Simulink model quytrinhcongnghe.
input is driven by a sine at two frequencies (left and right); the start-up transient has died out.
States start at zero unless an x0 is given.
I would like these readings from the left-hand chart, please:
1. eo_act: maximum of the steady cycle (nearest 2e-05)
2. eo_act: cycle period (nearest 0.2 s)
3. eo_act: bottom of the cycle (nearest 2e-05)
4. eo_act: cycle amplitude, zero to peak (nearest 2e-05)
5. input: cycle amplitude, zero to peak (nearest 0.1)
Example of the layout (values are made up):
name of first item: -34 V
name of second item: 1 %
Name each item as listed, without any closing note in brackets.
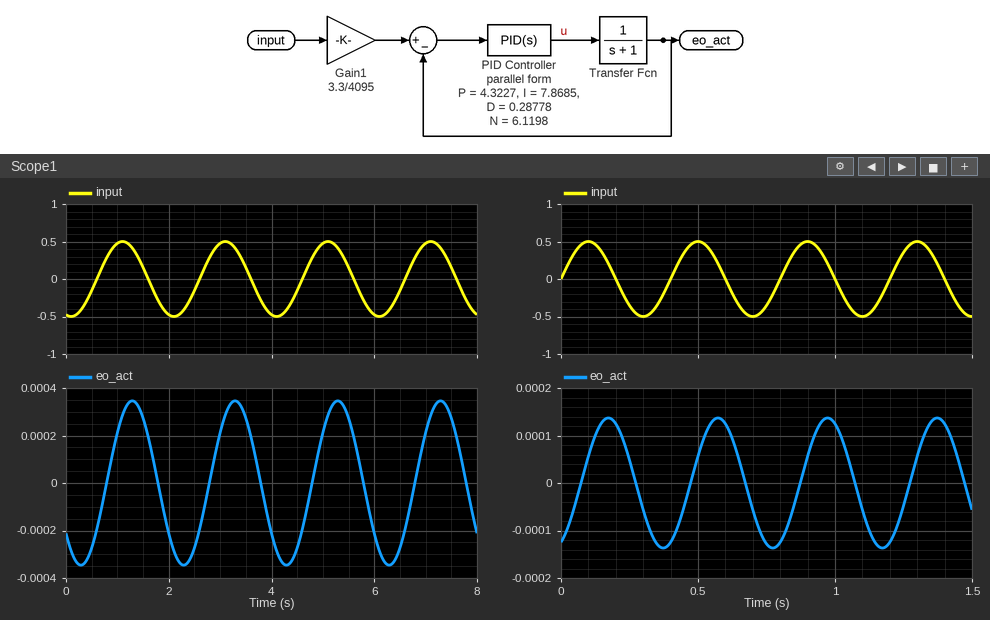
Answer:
eo_act: maximum of the steady cycle: 0.00034
eo_act: cycle period: 2.0 s
eo_act: bottom of the cycle: -0.00034
eo_act: cycle amplitude, zero to peak: 0.00034
input: cycle amplitude, zero to peak: 0.5
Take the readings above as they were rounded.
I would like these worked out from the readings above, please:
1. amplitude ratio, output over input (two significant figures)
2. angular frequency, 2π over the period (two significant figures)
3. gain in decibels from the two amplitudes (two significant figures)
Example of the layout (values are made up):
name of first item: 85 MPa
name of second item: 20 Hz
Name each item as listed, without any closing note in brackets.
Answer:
amplitude ratio, output over input: 0.00068
angular frequency, 2π over the period: 3.1 rad/s
gain in decibels from the two amplitudes: -63 dB
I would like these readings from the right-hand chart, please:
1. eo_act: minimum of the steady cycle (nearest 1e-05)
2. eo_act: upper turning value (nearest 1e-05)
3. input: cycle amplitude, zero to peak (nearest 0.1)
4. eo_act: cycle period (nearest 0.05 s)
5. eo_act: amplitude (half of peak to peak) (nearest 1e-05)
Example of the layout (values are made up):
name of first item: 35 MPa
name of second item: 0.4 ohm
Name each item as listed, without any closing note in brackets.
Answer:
eo_act: minimum of the steady cycle: -0.00014
eo_act: upper turning value: 0.00014
input: cycle amplitude, zero to peak: 0.5
eo_act: cycle period: 0.40 s
eo_act: amplitude (half of peak to peak): 0.00014
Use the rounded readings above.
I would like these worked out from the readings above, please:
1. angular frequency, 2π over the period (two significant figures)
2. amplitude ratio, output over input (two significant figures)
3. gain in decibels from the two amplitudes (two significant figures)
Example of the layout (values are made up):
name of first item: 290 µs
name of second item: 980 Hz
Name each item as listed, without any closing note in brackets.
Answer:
angular frequency, 2π over the period: 16 rad/s
amplitude ratio, output over input: 0.00028
gain in decibels from the two amplitudes: -71 dB
